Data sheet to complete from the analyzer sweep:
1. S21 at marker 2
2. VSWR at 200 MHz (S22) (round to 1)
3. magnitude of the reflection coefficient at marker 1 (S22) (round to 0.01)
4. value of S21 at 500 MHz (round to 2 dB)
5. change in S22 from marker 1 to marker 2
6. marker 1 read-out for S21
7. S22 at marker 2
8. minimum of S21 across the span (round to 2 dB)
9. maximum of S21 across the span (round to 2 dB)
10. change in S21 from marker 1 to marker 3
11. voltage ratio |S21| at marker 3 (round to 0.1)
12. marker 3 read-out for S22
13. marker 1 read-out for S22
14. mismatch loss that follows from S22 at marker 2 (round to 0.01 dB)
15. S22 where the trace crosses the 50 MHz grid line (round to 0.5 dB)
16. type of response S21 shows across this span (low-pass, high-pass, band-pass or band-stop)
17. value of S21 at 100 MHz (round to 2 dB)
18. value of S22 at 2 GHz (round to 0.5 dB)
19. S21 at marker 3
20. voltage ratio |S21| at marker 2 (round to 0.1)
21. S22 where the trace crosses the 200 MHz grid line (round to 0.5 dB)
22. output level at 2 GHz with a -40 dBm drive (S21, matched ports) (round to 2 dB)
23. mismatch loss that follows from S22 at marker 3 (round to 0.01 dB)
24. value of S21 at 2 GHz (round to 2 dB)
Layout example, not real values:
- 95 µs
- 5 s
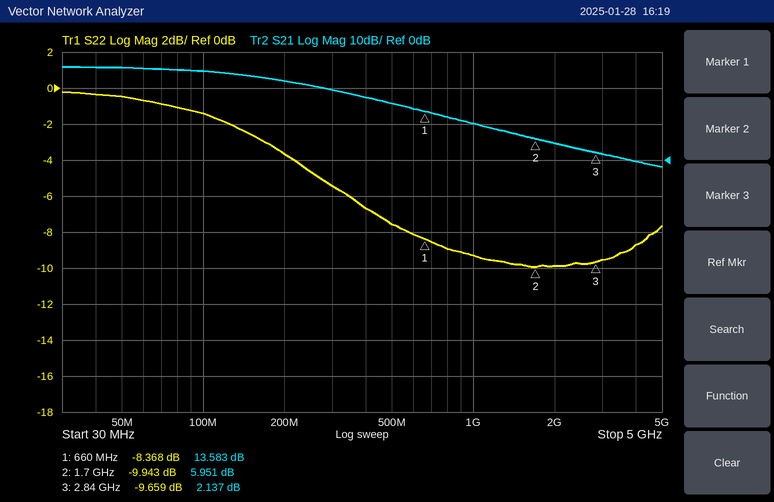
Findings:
- 5.951 dB
- 5
- 0.38
- 16 dB
- -1.575 dB
- 13.583 dB
- -9.943 dB
- -2 dB
- 26 dB
- -11.446 dB
- 1.3
- -9.659 dB
- -8.368 dB
- 0.46 dB
- -0.5 dB
- low-pass
- 24 dB
- -10.0 dB
- 2.137 dB
- 2.0
- -3.5 dB
- -36 dBm
- 0.50 dB
- 4 dB
